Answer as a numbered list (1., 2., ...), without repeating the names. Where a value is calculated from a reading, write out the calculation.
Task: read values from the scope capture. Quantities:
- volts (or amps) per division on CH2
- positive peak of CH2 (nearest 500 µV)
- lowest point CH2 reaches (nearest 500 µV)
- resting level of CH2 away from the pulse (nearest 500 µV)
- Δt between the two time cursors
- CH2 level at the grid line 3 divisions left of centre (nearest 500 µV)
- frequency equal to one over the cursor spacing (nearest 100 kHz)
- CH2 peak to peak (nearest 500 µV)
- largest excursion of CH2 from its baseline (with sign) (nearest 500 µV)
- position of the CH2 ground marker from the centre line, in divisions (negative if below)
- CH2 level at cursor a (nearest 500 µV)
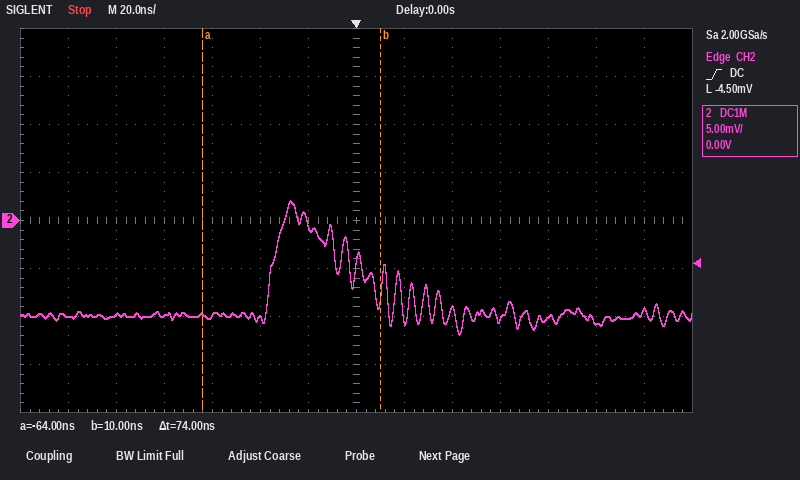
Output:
1. 5 mV
2. 2.0 mV
3. -12.0 mV
4. -10.0 mV
5. 74 ns
6. -10.0 mV
7. 1 / 74 ns ≈ 13.5 MHz
8. 2.0 mV − (-12.0 mV) = 14.0 mV
9. 2.0 mV − (-10.0 mV) = +12.0 mV
10. 0.0 div
11. -10.0 mV
